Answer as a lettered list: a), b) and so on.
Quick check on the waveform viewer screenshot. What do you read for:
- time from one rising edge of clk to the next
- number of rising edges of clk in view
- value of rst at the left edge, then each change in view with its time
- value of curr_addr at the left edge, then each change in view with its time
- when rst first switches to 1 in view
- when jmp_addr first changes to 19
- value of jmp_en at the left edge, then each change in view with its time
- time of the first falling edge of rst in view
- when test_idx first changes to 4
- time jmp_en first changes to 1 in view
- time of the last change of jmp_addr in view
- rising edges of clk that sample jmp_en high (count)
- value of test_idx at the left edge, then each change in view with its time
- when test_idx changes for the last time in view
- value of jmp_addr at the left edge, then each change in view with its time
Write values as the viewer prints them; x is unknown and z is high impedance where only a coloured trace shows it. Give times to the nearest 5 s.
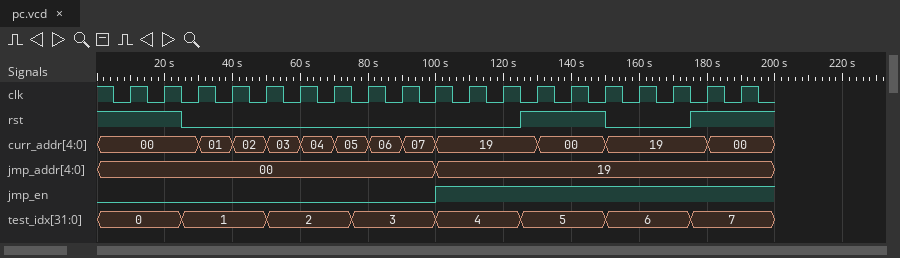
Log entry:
a) 10 s
b) 19
c) 1, 0 at 25 s, 1 at 125 s, 0 at 150 s, 1 at 175 s
d) 00, 01 at 30 s, 02 at 40 s, 03 at 50 s, 04 at 60 s, 05 at 70 s, 06 at 80 s, 07 at 90 s, 19 at 100 s, 00 at 130 s, 19 at 150 s, 00 at 180 s
e) 125 s
f) 100 s
g) 0, 1 at 100 s
h) 25 s
i) 100 s
j) 100 s
k) 100 s
l) 9
m) 0, 1 at 25 s, 2 at 50 s, 3 at 75 s, 4 at 100 s, 5 at 125 s, 6 at 150 s, 7 at 175 s
n) 175 s
o) 00, 19 at 100 s
